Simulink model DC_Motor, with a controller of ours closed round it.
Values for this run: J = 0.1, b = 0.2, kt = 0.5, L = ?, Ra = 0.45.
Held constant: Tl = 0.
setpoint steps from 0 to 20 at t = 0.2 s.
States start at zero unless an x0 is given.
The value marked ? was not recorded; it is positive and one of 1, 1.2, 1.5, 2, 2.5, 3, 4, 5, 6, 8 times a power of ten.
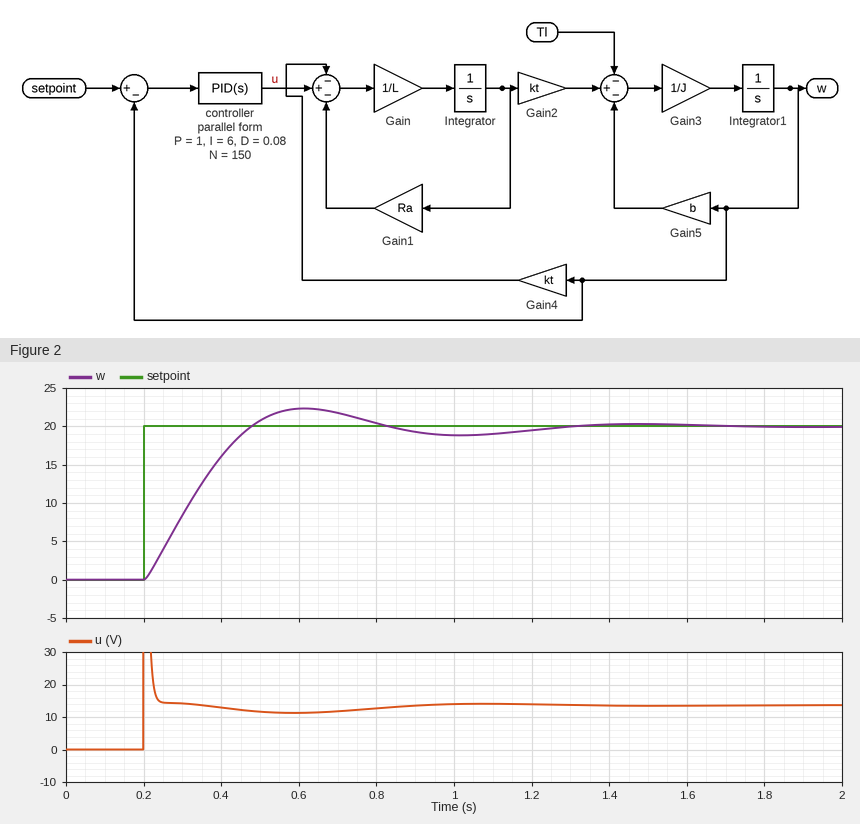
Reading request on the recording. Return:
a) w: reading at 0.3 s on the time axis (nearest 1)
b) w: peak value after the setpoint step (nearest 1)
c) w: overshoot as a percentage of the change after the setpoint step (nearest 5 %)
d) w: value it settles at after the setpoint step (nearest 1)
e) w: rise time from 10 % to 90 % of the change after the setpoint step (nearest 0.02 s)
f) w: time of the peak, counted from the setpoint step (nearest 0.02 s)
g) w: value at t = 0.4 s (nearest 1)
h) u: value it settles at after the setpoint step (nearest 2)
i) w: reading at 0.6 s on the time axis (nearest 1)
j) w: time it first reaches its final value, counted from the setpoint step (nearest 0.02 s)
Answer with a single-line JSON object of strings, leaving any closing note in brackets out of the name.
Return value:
{"w: reading at 0.3 s on the time axis": "8", "w: peak value after the setpoint step": "22", "w: overshoot as a percentage of the change after the setpoint step": "10 %", "w: value it settles at after the setpoint step": "20", "w: rise time from 10 % to 90 % of the change after the setpoint step": "0.20 s", "w: time of the peak, counted from the setpoint step": "0.42 s", "w: value at t = 0.4 s": "16", "u: value it settles at after the setpoint step": "14", "w: reading at 0.6 s on the time axis": "22", "w: time it first reaches its final value, counted from the setpoint step": "0.28 s"}
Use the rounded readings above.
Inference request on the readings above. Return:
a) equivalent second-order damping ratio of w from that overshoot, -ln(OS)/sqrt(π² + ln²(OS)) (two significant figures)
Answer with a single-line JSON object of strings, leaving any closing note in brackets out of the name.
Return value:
{"equivalent second-order damping ratio of w from that overshoot, -ln(OS)/sqrt(π² + ln²(OS))": "0.59"}
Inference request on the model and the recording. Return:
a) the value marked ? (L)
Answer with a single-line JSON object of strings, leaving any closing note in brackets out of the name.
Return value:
{"the value marked ?": "0.1"}
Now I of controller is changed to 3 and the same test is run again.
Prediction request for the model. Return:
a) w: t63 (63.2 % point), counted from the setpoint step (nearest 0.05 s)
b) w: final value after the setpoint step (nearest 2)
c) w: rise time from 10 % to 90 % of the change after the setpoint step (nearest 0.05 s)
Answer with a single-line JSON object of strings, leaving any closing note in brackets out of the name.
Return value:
{"w: t63 (63.2 % point), counted from the setpoint step": "0.15 s", "w: final value after the setpoint step": "20", "w: rise time from 10 % to 90 % of the change after the setpoint step": "0.30 s"}
